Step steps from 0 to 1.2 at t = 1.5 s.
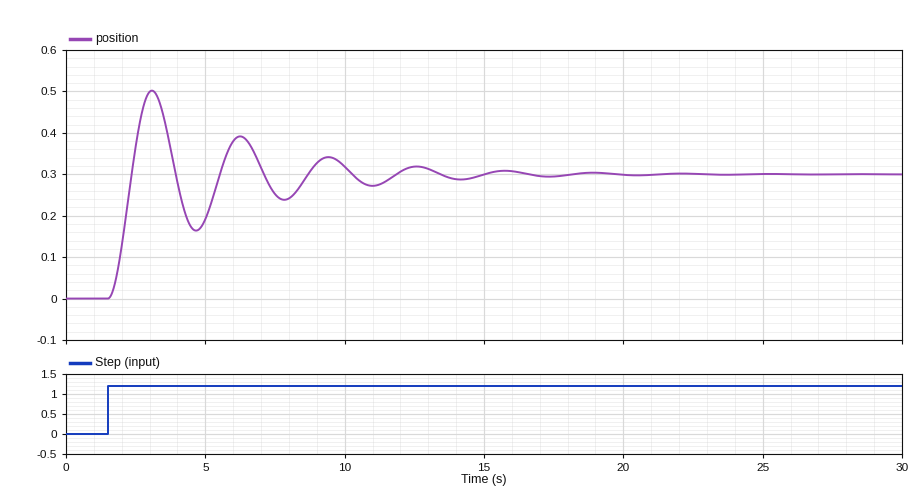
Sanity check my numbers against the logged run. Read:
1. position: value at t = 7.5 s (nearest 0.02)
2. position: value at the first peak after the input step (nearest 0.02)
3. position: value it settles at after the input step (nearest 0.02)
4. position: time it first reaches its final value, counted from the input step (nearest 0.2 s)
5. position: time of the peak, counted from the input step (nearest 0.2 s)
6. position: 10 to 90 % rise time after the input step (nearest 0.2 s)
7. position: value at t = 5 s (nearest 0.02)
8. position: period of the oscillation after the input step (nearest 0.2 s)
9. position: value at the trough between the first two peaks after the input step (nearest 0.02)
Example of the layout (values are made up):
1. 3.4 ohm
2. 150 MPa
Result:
1. 0.26
2. 0.50
3. 0.30
4. 0.8 s
5. 1.6 s
6. 0.6 s
7. 0.20
8. 3.2 s
9. 0.16
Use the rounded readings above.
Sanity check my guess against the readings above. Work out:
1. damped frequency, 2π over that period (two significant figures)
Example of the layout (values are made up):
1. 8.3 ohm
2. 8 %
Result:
1. 2.0 rad/s
